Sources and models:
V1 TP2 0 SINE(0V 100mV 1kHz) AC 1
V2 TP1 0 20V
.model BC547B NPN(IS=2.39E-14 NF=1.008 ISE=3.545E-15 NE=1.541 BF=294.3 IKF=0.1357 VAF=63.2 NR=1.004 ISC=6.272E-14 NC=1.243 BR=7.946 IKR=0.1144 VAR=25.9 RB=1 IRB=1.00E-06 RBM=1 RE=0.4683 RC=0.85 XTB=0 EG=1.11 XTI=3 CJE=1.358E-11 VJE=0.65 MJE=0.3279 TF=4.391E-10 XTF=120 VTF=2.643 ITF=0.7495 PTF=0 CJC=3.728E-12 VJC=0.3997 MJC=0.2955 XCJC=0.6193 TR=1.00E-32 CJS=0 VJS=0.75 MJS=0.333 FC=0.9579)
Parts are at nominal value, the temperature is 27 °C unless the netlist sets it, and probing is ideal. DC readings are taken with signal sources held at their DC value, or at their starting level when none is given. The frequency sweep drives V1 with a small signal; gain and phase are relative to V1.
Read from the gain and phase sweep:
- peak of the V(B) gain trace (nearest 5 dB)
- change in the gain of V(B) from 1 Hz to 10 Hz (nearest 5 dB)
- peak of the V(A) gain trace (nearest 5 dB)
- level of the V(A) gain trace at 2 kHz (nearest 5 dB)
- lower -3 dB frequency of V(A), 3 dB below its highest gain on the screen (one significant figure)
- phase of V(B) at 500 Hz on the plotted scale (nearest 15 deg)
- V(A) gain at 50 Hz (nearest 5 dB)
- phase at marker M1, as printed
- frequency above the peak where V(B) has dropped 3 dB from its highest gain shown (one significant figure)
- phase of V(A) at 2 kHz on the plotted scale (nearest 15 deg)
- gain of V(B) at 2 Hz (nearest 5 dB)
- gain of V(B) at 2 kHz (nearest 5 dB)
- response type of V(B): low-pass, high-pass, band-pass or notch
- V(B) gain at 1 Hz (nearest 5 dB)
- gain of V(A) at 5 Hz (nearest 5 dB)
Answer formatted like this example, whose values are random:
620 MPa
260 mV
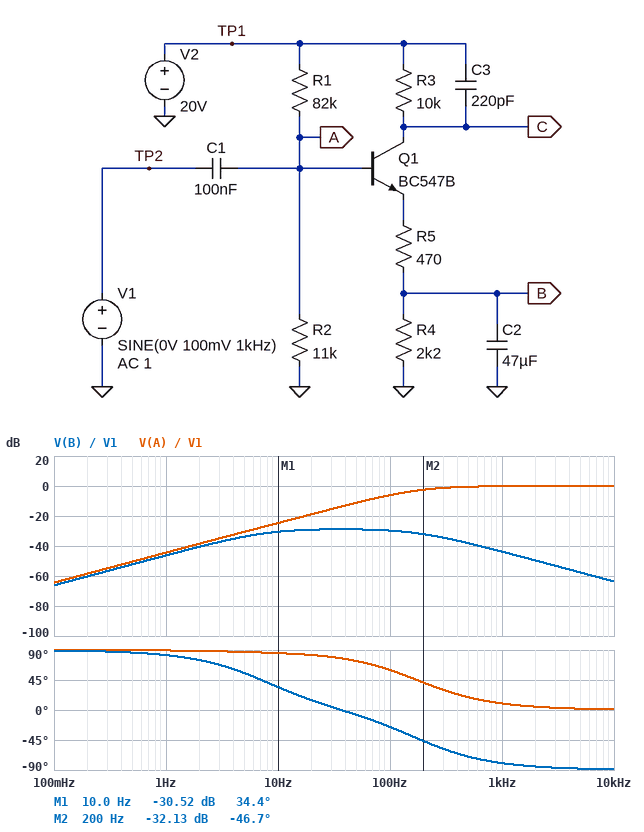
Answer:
-30 dB
15 dB
0 dB
0 dB
200 Hz
-75 deg
-10 dB
34.4 deg
200 Hz
0 deg
-40 dB
-50 dB
band-pass
-45 dB
-30 dB
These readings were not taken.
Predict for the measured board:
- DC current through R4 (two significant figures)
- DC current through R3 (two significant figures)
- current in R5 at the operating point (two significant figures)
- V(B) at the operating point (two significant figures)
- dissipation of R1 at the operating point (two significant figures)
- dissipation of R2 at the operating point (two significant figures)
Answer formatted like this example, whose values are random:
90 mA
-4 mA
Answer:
650 µA
640 µA
650 µA
1.4 V
3.8 mW
500 µW
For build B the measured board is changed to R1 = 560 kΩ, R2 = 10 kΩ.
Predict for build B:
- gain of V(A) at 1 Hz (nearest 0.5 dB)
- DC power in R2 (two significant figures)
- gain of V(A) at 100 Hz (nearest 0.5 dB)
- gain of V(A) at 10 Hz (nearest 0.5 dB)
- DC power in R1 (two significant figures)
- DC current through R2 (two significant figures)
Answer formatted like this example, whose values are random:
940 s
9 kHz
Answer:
-44.0 dB
12 µW
-5.5 dB
-24.0 dB
690 µW
35 µA
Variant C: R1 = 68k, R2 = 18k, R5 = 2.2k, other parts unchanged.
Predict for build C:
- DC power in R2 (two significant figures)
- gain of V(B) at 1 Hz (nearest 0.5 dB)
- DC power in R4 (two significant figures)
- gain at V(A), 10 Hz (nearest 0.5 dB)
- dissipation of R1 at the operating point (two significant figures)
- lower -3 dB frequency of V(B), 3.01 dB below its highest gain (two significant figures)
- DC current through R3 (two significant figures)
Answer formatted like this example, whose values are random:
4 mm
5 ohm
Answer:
960 µW
-47.5 dB
1.4 mW
-21.0 dB
3.7 mW
2.9 Hz
800 µA
